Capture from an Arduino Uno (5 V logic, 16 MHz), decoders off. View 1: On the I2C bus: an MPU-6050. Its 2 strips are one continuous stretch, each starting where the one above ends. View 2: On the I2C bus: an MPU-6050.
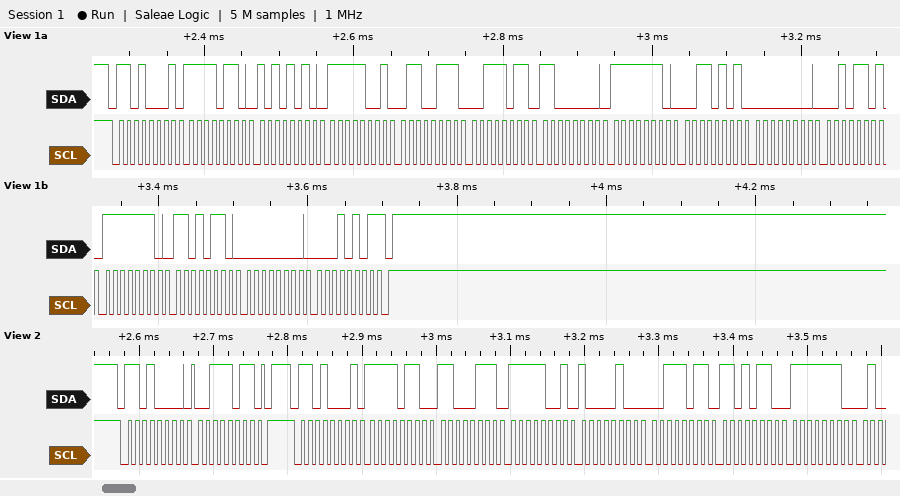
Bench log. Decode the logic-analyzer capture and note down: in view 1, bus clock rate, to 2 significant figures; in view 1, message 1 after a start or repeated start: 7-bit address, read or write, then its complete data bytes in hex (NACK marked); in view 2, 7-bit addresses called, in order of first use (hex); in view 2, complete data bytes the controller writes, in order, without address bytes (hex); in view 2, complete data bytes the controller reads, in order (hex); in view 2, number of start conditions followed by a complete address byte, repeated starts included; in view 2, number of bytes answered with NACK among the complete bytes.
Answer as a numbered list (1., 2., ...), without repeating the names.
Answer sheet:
1. 100 kHz
2. 0x68 read: F6 AA F9 67 3B C0 FE 35 00 2D FE D6 00 15 NACK
3. 0x68
4. 3B
5. F6 C7 F9 84 3B D6 FE
6. 2
7. 0
